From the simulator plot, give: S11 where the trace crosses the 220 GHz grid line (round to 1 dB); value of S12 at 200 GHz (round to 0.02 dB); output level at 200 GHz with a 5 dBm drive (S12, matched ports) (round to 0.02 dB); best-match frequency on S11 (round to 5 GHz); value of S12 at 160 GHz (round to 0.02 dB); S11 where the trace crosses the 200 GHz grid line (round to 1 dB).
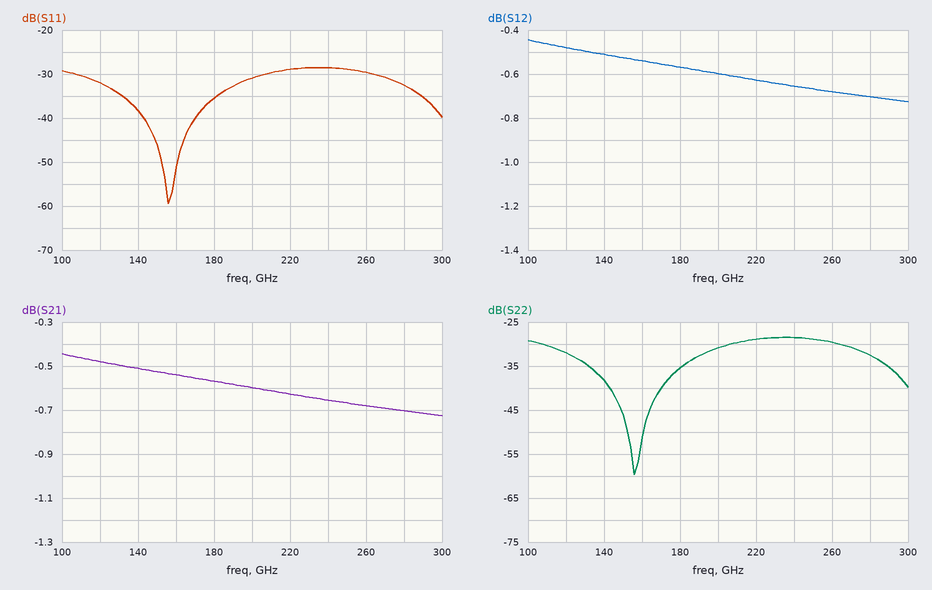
-29 dB
-0.60 dB
4.40 dBm
155 GHz
-0.54 dB
-31 dB
